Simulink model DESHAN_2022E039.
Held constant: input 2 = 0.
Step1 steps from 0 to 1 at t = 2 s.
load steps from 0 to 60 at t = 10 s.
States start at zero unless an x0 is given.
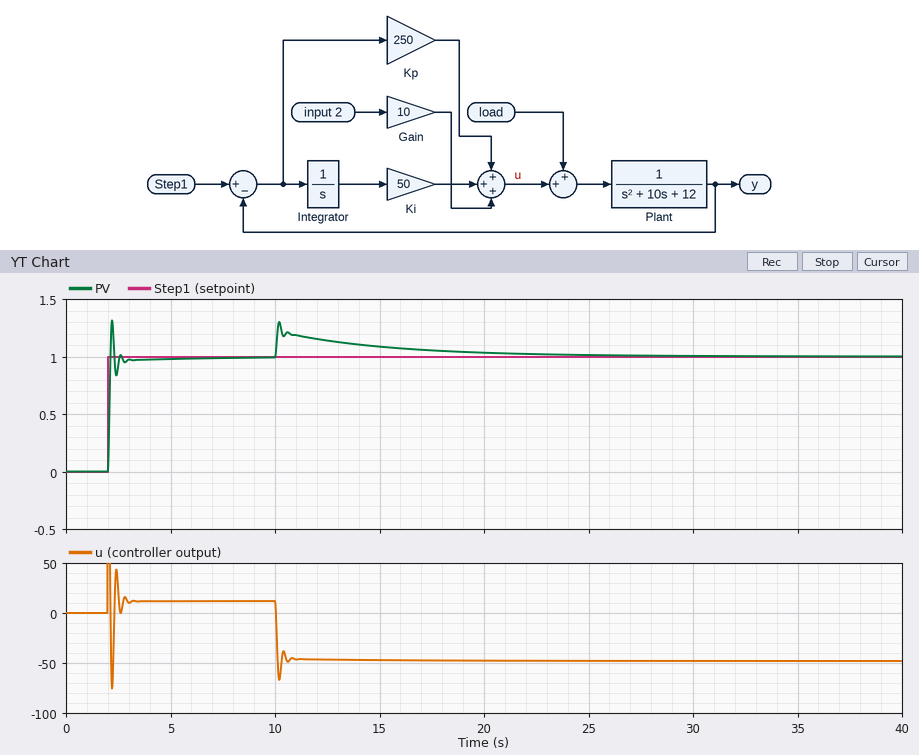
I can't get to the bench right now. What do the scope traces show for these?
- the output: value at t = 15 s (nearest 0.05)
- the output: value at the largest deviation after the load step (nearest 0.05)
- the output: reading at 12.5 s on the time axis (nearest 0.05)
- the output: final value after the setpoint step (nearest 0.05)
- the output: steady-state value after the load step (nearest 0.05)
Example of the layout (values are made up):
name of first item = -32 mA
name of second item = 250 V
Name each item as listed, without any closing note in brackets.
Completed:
the output: value at t = 15 s = 1.10
the output: value at the largest deviation after the load step = 1.30
the output: reading at 12.5 s on the time axis = 1.15
the output: final value after the setpoint step = 1.00
the output: steady-state value after the load step = 1.00
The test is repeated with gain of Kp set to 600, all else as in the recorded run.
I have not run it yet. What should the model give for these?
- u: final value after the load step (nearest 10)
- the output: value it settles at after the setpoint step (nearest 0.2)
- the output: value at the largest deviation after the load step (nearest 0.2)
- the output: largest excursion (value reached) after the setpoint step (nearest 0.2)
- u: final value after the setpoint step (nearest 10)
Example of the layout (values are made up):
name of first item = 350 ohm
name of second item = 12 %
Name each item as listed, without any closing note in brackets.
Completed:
u: final value after the load step = -50
the output: value it settles at after the setpoint step = 1.0
the output: value at the largest deviation after the load step = 1.2
the output: largest excursion (value reached) after the setpoint step = 1.4
u: final value after the setpoint step = 10
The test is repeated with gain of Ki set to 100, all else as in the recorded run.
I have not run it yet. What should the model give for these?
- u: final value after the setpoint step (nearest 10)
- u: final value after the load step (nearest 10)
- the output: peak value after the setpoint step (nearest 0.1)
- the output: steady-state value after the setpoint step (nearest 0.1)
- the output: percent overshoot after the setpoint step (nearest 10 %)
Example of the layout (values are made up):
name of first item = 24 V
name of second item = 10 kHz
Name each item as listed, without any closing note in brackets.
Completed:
u: final value after the setpoint step = 10
u: final value after the load step = -50
the output: peak value after the setpoint step = 1.3
the output: steady-state value after the setpoint step = 1.0
the output: percent overshoot after the setpoint step = 30 %
